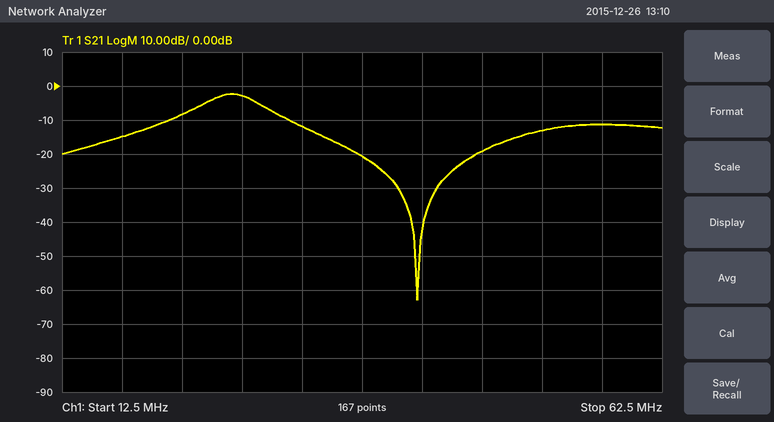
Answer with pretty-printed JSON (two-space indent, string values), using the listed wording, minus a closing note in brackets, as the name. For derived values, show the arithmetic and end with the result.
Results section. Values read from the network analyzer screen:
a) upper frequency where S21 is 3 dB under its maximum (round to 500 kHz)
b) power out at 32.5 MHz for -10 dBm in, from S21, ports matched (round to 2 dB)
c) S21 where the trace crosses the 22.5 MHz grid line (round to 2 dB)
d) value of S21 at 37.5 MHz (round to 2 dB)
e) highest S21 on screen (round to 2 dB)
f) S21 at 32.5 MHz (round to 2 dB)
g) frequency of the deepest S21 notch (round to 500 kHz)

{
  "upper frequency where S21 is 3 dB under its maximum": "29.0 MHz",
  "power out at 32.5 MHz for -10 dBm in, from S21, ports matched": "-10 dBm + (-12 dB) = -22 dBm",
  "S21 where the trace crosses the 22.5 MHz grid line": "-8 dB",
  "value of S21 at 37.5 MHz": "-20 dB",
  "highest S21 on screen": "-2 dB",
  "S21 at 32.5 MHz": "-12 dB",
  "frequency of the deepest S21 notch": "42.0 MHz"
}
